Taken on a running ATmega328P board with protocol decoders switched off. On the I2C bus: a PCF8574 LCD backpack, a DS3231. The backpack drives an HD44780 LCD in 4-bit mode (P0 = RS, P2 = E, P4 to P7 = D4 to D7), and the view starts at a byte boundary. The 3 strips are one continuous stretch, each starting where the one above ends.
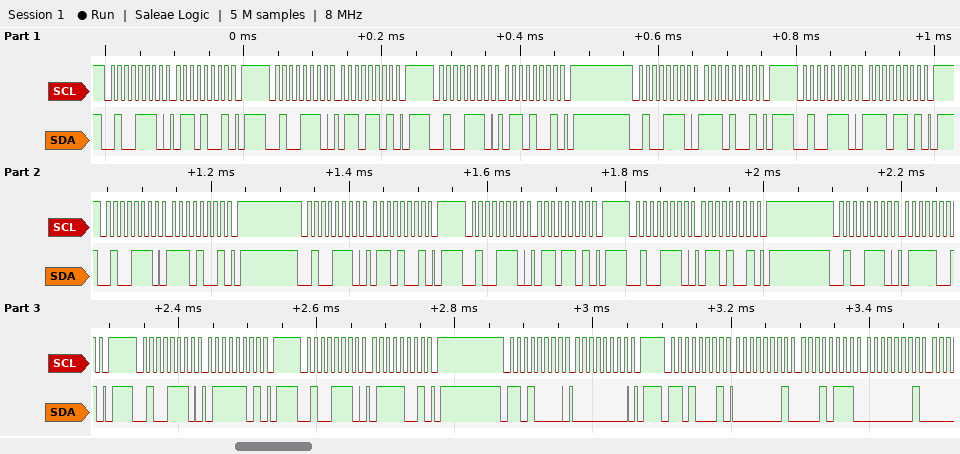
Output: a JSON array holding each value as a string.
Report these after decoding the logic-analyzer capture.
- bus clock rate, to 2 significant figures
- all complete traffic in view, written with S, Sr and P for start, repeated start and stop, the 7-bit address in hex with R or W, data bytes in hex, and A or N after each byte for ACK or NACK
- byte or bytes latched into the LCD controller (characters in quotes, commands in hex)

["100 kHz", "S 27W A 69 A P S 27W A 6D A P S 27W A 69 A P S 27W A E9 A P S 27W A ED A P S 27W A E9 A P S 27W A 69 A P S 27W A 6D A P S 27W A 69 A P S 27W A 79 A P S 27W A 7D A P S 27W A 79 A P S 68W A 00 A P S 68R A 01 A 17 A 01 A", "'n' 'g'"]
